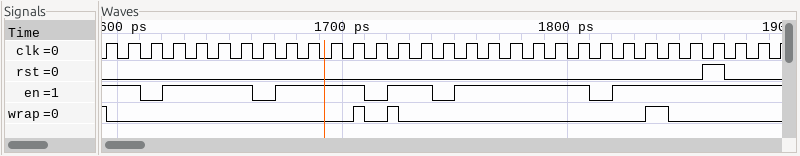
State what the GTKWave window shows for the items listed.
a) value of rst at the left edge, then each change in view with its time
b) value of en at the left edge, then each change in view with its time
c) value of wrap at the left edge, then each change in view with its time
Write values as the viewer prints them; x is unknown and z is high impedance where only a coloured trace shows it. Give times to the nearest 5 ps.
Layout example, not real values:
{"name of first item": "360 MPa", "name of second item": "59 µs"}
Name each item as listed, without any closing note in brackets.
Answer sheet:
{"value of rst at the left edge, then each change in view with its time": "0, 1 at 1860 ps, 0 at 1870 ps", "value of en at the left edge, then each change in view with its time": "1, 0 at 1610 ps, 1 at 1620 ps, 0 at 1660 ps, 1 at 1670 ps, 0 at 1710 ps, 1 at 1720 ps, 0 at 1740 ps, 1 at 1750 ps, 0 at 1810 ps, 1 at 1820 ps", "value of wrap at the left edge, then each change in view with its time": "1, 0 at 1595 ps, 1 at 1705 ps, 0 at 1710 ps, 1 at 1720 ps, 0 at 1725 ps, 1 at 1835 ps, 0 at 1845 ps"}
